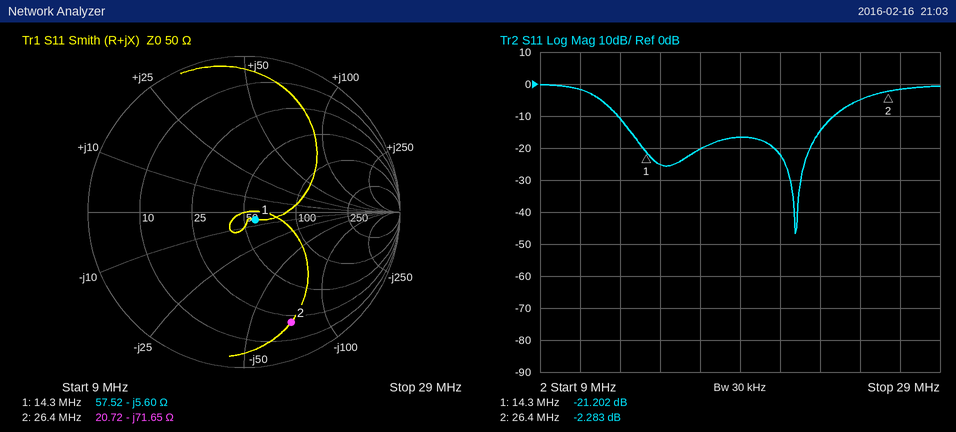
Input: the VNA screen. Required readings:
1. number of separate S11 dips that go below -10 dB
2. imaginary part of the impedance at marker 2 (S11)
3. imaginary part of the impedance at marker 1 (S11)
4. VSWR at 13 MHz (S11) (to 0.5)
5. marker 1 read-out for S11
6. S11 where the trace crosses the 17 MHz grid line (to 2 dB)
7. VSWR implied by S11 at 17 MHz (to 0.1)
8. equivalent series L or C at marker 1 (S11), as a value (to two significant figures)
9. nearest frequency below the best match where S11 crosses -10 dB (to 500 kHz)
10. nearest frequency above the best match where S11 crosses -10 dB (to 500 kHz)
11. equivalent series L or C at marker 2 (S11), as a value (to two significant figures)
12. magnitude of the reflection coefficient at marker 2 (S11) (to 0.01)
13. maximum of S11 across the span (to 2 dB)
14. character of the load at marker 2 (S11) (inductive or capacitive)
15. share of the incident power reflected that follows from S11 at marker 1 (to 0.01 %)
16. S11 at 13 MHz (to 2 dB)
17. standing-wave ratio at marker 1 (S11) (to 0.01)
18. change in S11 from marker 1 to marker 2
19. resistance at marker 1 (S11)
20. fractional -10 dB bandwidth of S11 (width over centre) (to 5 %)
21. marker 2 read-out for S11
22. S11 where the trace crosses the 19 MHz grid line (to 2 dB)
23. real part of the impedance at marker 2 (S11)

2
-71.65 Ω
-5.60 Ω
2.0
-21.202 dB
-20 dB
1.2
2.0 nF
13.0 MHz
23.5 MHz
84 pF
0.77
0 dB
capacitive
0.76 %
-10 dB
1.19
18.919 dB
57.52 Ω
60 %
-2.283 dB
-16 dB
20.72 Ω
